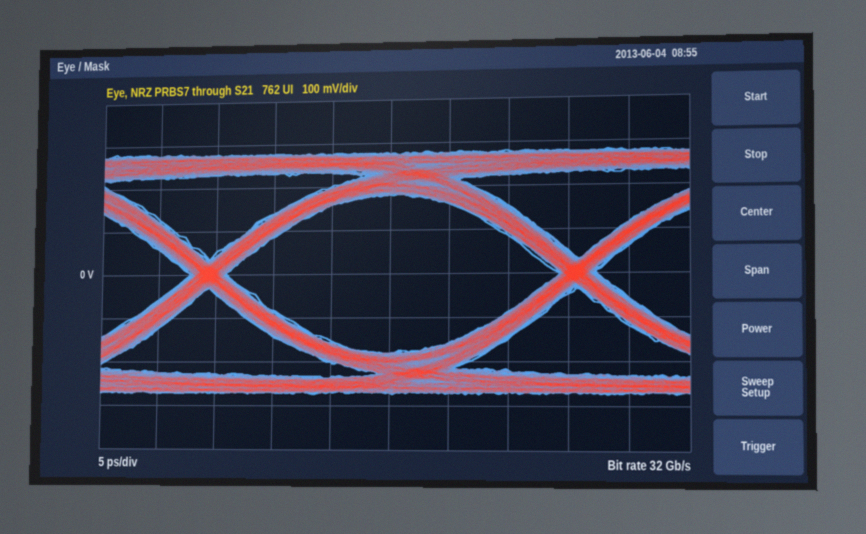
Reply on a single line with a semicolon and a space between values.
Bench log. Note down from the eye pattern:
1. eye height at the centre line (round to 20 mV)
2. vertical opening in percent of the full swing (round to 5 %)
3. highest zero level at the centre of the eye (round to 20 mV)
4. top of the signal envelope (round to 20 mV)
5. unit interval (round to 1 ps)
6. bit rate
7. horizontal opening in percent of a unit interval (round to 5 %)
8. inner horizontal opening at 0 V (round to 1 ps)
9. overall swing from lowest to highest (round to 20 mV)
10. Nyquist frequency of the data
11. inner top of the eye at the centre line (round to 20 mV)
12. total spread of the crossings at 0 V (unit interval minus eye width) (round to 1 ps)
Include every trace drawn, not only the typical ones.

360 mV; 65 %; -180 mV; 280 mV; 31 ps; 32 Gb/s; 90 %; 28 ps; 560 mV; 16 GHz; 180 mV; 3 ps
